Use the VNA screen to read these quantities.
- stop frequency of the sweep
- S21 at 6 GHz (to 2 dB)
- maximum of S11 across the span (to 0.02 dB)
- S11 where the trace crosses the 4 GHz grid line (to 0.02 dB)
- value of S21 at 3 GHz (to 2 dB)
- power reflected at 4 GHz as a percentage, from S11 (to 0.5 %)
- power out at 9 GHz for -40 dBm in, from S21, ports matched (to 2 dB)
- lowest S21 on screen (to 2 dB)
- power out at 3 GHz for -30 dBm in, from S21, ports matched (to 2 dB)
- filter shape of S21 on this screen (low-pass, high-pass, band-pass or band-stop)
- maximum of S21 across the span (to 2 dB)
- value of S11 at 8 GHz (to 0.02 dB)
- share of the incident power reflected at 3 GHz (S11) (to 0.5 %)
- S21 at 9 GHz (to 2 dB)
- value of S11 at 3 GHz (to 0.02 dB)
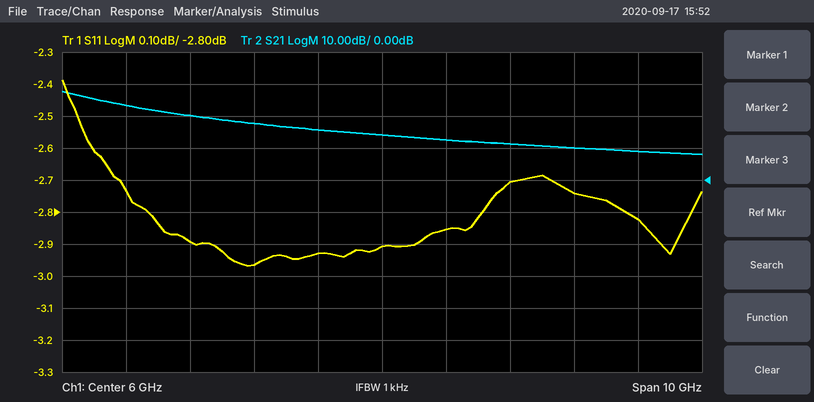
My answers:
11 GHz
14 dB
-2.38 dB
-2.96 dB
20 dB
50.5 %
-30 dBm
8 dB
-10 dBm
low-pass
28 dB
-2.70 dB
51.5 %
10 dB
-2.90 dB
